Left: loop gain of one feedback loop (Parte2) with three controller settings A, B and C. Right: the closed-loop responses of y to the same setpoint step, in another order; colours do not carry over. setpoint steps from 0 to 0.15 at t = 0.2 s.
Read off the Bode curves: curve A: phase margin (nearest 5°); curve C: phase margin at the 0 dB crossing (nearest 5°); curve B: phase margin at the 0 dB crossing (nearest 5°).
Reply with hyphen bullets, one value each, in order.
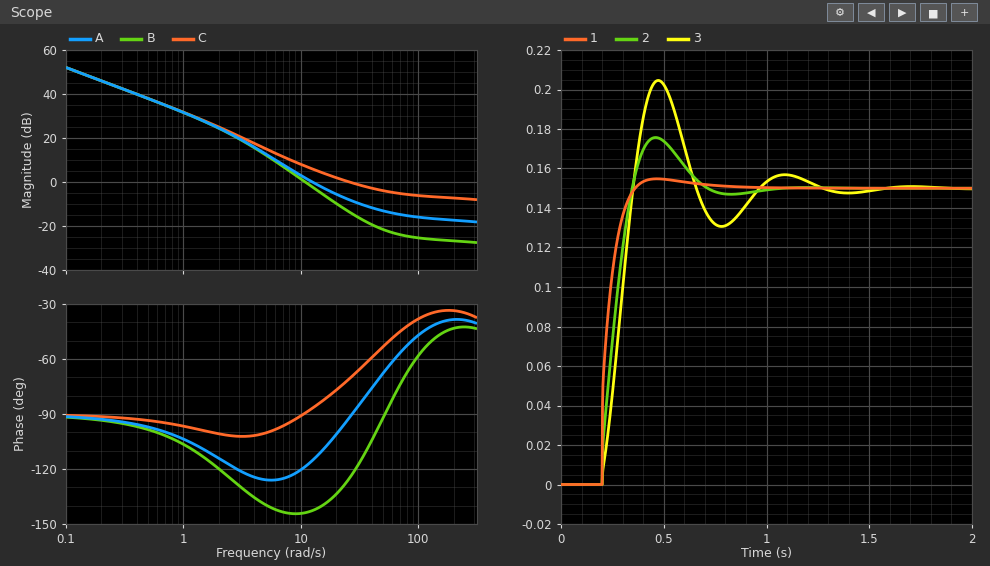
- 65°
- 110°
- 35°
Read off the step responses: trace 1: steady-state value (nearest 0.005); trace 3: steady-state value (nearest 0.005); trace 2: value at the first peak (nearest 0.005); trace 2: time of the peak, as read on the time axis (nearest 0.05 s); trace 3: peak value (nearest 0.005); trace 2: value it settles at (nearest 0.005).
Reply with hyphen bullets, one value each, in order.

- 0.150
- 0.150
- 0.175
- 0.45 s
- 0.205
- 0.150
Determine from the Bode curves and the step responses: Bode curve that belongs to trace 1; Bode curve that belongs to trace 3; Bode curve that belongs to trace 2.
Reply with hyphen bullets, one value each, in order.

- C
- B
- A
